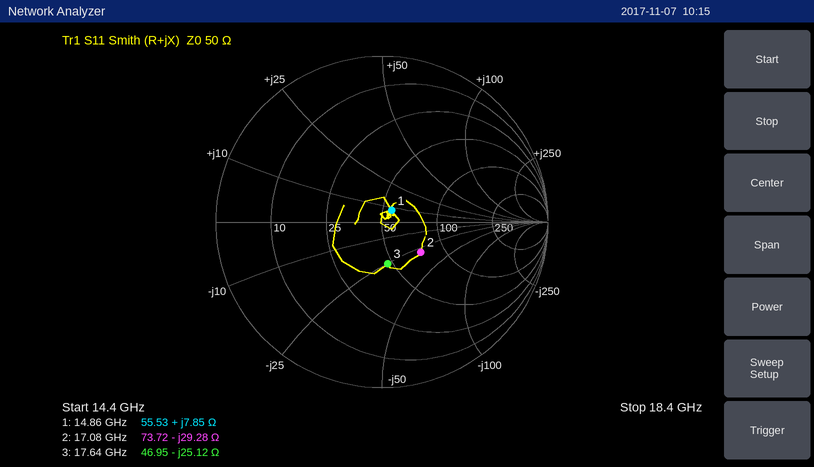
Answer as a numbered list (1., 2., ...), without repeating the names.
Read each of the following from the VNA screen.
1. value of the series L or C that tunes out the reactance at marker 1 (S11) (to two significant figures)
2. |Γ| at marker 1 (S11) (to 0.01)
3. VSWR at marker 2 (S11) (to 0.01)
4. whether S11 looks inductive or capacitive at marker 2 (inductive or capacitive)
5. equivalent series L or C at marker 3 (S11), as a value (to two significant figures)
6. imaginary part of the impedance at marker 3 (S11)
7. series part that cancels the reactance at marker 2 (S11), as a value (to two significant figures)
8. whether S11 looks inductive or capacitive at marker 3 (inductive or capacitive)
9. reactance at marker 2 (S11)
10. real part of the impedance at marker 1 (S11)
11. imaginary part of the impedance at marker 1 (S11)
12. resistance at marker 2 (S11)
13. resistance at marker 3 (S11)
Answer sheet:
1. 1.4 pF
2. 0.09
3. 1.84
4. capacitive
5. 360 fF
6. -25.12 Ω
7. 270 pH
8. capacitive
9. -29.28 Ω
10. 55.53 Ω
11. +7.85 Ω
12. 73.72 Ω
13. 46.95 Ω
